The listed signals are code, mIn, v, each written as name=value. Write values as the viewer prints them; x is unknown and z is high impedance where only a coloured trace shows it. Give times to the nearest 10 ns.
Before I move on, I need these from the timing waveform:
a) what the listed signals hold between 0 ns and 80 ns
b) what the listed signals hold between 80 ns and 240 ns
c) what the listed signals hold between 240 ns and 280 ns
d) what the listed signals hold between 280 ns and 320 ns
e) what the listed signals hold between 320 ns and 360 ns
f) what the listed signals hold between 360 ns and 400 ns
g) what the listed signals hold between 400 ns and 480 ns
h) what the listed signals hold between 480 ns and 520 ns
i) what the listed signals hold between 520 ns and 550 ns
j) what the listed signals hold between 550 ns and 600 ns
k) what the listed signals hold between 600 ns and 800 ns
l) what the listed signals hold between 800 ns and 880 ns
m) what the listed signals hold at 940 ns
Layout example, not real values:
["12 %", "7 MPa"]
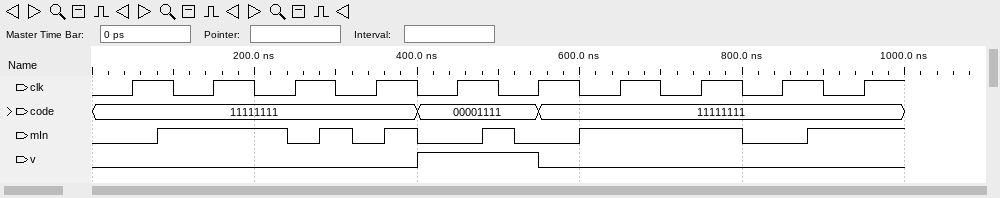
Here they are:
["code=11111111, mIn=0, v=0", "code=11111111, mIn=1, v=0", "code=11111111, mIn=0, v=0", "code=11111111, mIn=1, v=0", "code=11111111, mIn=0, v=0", "code=11111111, mIn=1, v=0", "code=00001111, mIn=0, v=1", "code=00001111, mIn=1, v=1", "code=00001111, mIn=0, v=1", "code=11111111, mIn=0, v=0", "code=11111111, mIn=1, v=0", "code=11111111, mIn=0, v=0", "code=11111111, mIn=1, v=0"]
